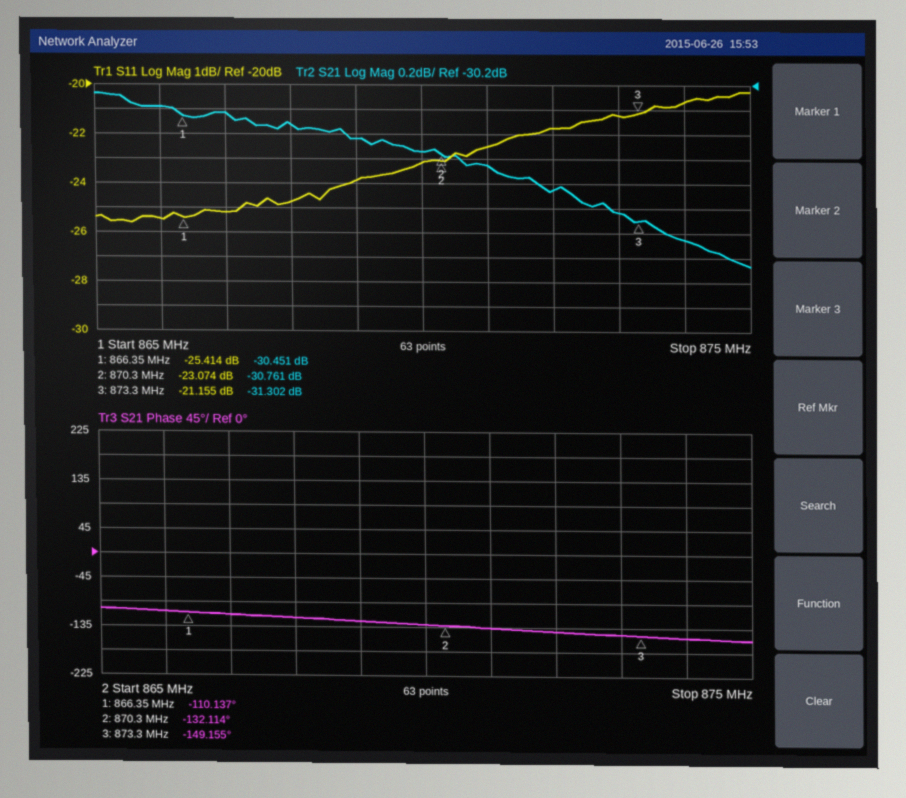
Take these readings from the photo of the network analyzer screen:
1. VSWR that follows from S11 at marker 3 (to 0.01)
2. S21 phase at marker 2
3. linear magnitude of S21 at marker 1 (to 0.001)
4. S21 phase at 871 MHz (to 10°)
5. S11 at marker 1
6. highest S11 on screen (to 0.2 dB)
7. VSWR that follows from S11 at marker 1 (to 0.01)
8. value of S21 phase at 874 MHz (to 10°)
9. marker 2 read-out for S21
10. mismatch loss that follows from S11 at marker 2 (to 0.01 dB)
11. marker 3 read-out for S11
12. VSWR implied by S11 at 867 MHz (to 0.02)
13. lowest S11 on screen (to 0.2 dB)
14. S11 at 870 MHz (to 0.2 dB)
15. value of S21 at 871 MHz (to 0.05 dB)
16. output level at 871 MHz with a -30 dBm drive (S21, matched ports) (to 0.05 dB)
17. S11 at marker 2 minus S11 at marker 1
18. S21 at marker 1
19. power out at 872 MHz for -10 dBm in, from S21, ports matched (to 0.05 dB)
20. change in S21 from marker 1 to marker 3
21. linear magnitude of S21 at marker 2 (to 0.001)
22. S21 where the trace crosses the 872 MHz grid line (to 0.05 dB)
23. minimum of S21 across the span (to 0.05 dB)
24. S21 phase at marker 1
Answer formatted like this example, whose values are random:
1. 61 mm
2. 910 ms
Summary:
1. 1.19
2. -132.114°
3. 0.030
4. -140°
5. -25.414 dB
6. -20.2 dB
7. 1.11
8. -150°
9. -30.761 dB
10. 0.02 dB
11. -21.155 dB
12. 1.12
13. -25.6 dB
14. -23.2 dB
15. -30.85 dB
16. -60.85 dBm
17. 2.340 dB
18. -30.451 dB
19. -41.05 dBm
20. -0.851 dB
21. 0.029
22. -31.05 dB
23. -31.65 dB
24. -110.137°
